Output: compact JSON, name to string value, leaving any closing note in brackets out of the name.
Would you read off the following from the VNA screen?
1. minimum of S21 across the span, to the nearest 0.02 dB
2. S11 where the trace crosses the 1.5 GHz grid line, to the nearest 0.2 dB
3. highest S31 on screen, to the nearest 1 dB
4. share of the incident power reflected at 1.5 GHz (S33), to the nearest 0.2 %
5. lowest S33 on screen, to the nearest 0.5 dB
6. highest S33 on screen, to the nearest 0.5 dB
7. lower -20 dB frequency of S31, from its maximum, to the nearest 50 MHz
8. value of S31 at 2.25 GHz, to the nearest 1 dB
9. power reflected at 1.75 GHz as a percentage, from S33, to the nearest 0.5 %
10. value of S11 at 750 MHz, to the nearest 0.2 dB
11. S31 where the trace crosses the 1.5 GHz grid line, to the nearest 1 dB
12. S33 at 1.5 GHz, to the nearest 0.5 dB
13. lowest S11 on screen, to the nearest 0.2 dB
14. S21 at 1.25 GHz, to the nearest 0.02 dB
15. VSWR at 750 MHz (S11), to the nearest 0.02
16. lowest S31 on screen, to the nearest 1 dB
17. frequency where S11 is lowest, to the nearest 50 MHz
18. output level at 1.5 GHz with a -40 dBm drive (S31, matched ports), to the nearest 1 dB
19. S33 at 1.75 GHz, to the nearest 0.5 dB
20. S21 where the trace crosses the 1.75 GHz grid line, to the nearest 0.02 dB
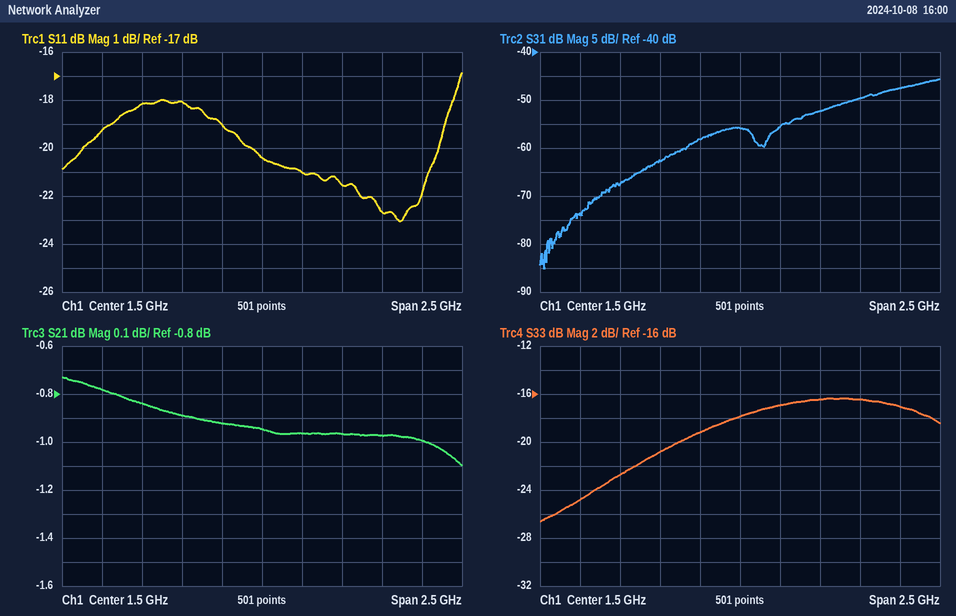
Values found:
{"minimum of S21 across the span, to the nearest 0.02 dB": "-1.10 dB", "S11 where the trace crosses the 1.5 GHz grid line, to the nearest 0.2 dB": "-20.4 dB", "highest S31 on screen, to the nearest 1 dB": "-46 dB", "share of the incident power reflected at 1.5 GHz (S33), to the nearest 0.2 %": "1.6 %", "lowest S33 on screen, to the nearest 0.5 dB": "-26.5 dB", "highest S33 on screen, to the nearest 0.5 dB": "-16.5 dB", "lower -20 dB frequency of S31, from its maximum, to the nearest 50 MHz": "850 MHz", "value of S31 at 2.25 GHz, to the nearest 1 dB": "-50 dB", "power reflected at 1.75 GHz as a percentage, from S33, to the nearest 0.5 %": "2.0 %", "value of S11 at 750 MHz, to the nearest 0.2 dB": "-18.2 dB", "S31 where the trace crosses the 1.5 GHz grid line, to the nearest 1 dB": "-56 dB", "S33 at 1.5 GHz, to the nearest 0.5 dB": "-18.0 dB", "lowest S11 on screen, to the nearest 0.2 dB": "-23.0 dB", "S21 at 1.25 GHz, to the nearest 0.02 dB": "-0.92 dB", "VSWR at 750 MHz (S11), to the nearest 0.02": "1.28", "lowest S31 on screen, to the nearest 1 dB": "-85 dB", "frequency where S11 is lowest, to the nearest 50 MHz": "2.35 GHz", "output level at 1.5 GHz with a -40 dBm drive (S31, matched ports), to the nearest 1 dB": "-96 dBm", "S33 at 1.75 GHz, to the nearest 0.5 dB": "-17.0 dB", "S21 where the trace crosses the 1.75 GHz grid line, to the nearest 0.02 dB": "-0.96 dB"}
